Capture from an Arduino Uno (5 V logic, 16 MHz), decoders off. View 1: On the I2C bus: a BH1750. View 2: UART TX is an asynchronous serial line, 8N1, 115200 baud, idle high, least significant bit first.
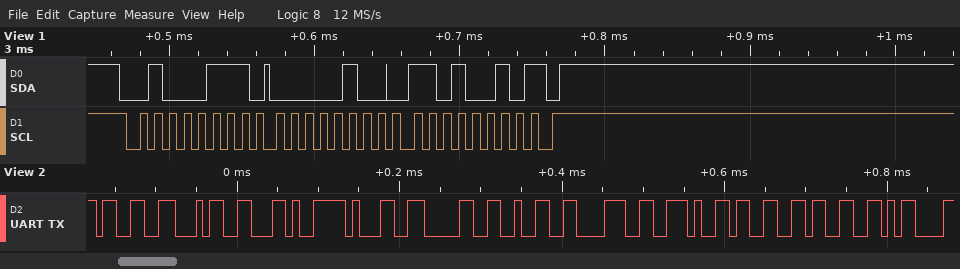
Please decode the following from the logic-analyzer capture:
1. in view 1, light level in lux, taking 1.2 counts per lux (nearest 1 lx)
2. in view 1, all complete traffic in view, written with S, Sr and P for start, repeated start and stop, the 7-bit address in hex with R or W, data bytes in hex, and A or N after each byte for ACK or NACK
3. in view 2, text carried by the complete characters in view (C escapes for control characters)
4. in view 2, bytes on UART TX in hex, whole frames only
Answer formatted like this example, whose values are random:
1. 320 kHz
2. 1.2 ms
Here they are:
1. 1028 lx
2. S 23R A 04 A D2 N P
3. "34,1028.33\r"
4. 33 34 2C 31 30 32 38 2E 33 33 0D
